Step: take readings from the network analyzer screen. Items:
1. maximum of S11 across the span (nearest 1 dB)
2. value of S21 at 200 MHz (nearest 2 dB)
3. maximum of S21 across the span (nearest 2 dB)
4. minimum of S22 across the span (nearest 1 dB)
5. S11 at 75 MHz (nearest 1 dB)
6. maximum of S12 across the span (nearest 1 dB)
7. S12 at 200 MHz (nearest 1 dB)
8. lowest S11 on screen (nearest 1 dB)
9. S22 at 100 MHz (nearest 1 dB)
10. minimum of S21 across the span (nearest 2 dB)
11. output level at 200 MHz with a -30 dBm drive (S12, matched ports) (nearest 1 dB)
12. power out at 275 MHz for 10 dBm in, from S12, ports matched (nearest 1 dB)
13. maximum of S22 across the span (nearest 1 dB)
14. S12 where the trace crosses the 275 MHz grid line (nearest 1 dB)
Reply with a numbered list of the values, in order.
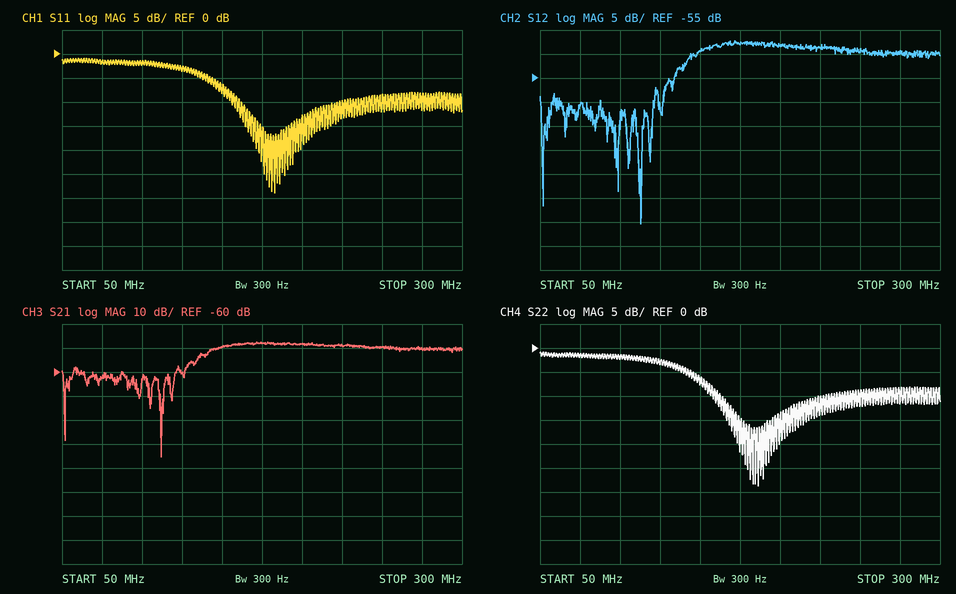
1. -1 dB
2. -48 dB
3. -48 dB
4. -29 dB
5. -2 dB
6. -47 dB
7. -48 dB
8. -29 dB
9. -2 dB
10. -96 dB
11. -78 dBm
12. -40 dBm
13. -1 dB
14. -50 dB
